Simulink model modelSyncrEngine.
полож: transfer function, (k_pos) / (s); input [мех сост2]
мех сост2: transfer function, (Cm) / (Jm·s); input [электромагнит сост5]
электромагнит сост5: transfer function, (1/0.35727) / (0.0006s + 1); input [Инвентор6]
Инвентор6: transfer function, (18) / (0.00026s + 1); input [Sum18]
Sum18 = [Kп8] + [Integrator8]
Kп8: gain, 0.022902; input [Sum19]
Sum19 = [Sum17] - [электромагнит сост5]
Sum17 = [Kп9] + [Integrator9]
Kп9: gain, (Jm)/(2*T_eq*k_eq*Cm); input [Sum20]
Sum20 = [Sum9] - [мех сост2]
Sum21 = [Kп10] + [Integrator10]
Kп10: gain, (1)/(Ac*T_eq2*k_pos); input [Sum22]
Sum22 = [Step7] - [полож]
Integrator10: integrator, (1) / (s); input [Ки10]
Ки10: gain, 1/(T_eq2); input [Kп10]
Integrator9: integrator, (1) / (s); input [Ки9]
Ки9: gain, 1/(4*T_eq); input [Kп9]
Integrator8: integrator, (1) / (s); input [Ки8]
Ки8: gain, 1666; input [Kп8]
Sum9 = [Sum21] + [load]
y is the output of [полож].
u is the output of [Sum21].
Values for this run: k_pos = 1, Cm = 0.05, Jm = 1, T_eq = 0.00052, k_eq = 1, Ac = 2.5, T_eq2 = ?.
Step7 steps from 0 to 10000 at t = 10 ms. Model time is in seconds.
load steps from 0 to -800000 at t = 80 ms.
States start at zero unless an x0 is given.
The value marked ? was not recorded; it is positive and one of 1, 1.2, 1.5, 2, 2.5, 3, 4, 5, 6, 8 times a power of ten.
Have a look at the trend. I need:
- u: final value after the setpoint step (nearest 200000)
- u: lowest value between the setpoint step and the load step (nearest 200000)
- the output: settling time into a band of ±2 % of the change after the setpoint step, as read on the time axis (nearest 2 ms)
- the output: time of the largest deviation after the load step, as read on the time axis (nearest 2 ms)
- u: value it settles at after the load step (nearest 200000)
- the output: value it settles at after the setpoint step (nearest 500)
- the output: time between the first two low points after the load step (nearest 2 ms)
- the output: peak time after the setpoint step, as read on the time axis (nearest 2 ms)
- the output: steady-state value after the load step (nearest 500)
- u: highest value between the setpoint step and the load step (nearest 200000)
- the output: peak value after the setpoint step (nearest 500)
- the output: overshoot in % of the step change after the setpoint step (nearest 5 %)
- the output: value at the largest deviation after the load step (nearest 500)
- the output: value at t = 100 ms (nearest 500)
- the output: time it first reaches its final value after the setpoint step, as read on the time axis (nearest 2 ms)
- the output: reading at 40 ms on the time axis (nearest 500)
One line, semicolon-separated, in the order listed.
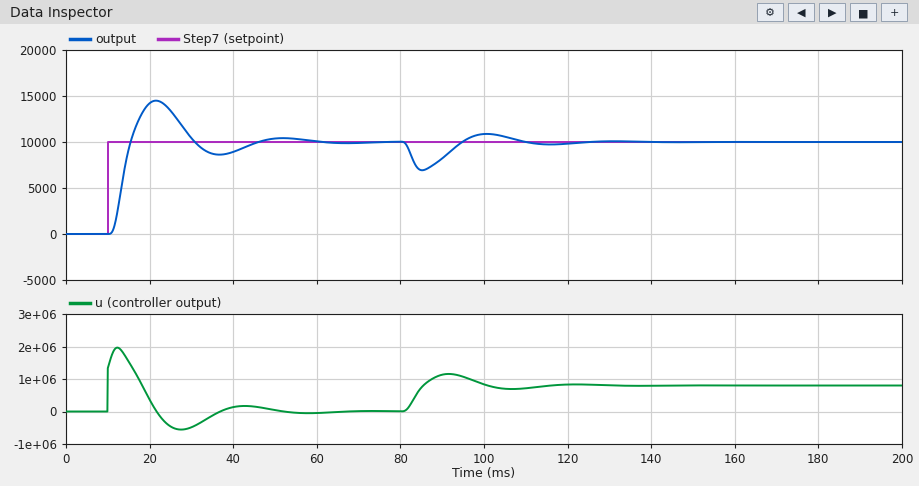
0; -600000; 58 ms; 86 ms; 800000; 10000; 30 ms; 22 ms; 10000; 2000000; 14500; 45 %; 7000; 11000; 16 ms; 9000
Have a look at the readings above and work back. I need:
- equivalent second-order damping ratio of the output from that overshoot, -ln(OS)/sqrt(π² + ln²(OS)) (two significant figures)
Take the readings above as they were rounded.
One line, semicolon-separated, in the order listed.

0.25
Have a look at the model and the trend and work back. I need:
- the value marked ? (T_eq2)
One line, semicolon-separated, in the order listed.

0.003
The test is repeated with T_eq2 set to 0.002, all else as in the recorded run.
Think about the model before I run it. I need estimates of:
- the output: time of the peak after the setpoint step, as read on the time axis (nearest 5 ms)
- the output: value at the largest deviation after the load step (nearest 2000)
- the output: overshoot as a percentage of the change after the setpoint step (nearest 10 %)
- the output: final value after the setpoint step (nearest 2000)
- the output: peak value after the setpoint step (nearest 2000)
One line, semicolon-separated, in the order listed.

15 ms; 8000; 60 %; 10000; 16000
